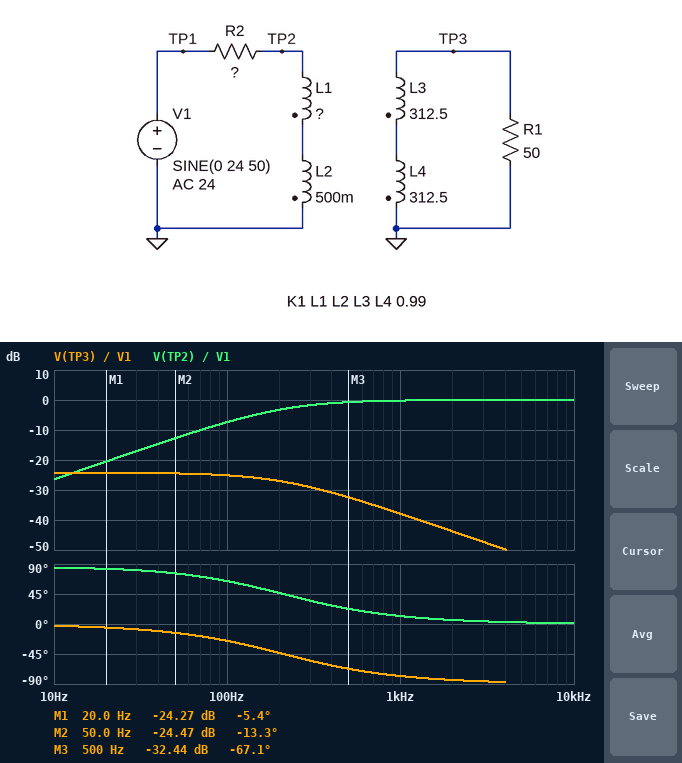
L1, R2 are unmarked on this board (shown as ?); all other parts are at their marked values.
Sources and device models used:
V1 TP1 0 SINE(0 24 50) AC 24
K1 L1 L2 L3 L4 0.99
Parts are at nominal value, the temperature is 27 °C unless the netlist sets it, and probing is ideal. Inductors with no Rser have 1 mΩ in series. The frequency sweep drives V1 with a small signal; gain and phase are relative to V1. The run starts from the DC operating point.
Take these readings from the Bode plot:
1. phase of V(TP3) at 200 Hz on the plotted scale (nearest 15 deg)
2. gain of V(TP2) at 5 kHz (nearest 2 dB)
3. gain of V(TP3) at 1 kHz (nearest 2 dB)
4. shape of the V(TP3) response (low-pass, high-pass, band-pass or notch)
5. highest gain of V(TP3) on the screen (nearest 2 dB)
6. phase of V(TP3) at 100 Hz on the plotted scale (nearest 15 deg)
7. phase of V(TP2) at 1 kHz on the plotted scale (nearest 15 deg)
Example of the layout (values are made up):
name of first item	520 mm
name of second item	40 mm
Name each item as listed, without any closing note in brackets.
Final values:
phase of V(TP3) at 200 Hz on the plotted scale	-45 deg
gain of V(TP2) at 5 kHz	0 dB
gain of V(TP3) at 1 kHz	-38 dB
shape of the V(TP3) response	low-pass
highest gain of V(TP3) on the screen	-24 dB
phase of V(TP3) at 100 Hz on the plotted scale	-30 deg
phase of V(TP2) at 1 kHz on the plotted scale	15 deg
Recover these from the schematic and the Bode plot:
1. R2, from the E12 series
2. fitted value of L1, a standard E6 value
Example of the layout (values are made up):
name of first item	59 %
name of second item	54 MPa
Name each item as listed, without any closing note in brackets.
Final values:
R2, from the E12 series	39 Ω
fitted value of L1, a standard E6 value	1 H
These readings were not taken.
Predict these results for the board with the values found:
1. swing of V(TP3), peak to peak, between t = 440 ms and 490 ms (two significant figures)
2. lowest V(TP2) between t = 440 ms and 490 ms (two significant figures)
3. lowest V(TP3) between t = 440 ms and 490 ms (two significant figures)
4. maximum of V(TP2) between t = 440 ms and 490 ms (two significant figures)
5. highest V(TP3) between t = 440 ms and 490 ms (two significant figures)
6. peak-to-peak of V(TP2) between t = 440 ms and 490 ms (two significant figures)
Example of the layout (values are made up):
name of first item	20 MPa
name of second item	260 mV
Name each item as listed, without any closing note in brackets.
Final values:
swing of V(TP3), peak to peak, between t = 440 ms and 490 ms	2.9 V
lowest V(TP2) between t = 440 ms and 490 ms	-5.5 V
lowest V(TP3) between t = 440 ms and 490 ms	-1.4 V
maximum of V(TP2) between t = 440 ms and 490 ms	5.5 V
highest V(TP3) between t = 440 ms and 490 ms	1.4 V
peak-to-peak of V(TP2) between t = 440 ms and 490 ms	11 V
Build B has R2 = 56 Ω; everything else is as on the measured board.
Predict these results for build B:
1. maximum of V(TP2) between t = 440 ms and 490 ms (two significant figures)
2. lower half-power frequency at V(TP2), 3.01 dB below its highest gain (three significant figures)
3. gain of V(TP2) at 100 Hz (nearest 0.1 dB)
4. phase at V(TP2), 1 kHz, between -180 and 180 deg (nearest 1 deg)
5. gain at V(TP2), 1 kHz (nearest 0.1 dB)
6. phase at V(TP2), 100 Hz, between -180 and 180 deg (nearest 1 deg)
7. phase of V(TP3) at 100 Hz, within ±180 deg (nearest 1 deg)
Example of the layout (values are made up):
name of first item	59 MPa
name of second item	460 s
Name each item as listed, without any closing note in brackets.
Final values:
maximum of V(TP2) between t = 440 ms and 490 ms	3.9 V
lower half-power frequency at V(TP2), 3.01 dB below its highest gain	303 Hz
gain of V(TP2) at 100 Hz	-10.1 dB
phase at V(TP2), 1 kHz, between -180 and 180 deg	17 deg
gain at V(TP2), 1 kHz	-0.4 dB
phase at V(TP2), 100 Hz, between -180 and 180 deg	71 deg
phase of V(TP3) at 100 Hz, within ±180 deg	-18 deg
